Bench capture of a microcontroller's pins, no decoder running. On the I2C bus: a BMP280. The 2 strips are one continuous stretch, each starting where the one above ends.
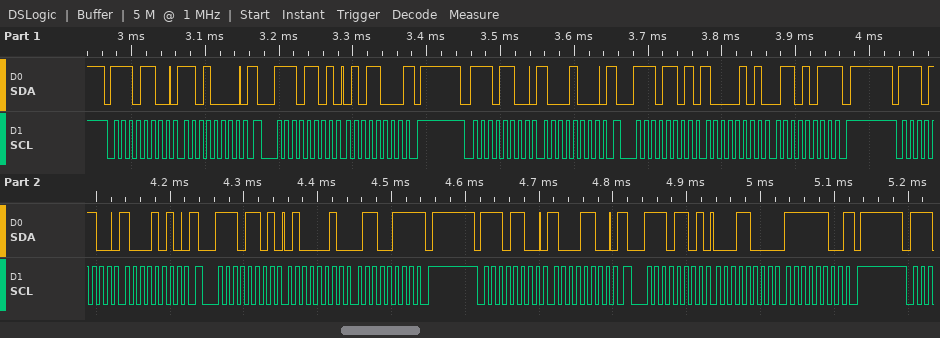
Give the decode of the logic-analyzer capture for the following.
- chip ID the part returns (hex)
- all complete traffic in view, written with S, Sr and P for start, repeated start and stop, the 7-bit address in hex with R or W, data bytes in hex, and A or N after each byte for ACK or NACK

0x58
S 76W A D0 A Sr 76R A 58 N P S 76W A 88 A Sr 76R A 85 A 6B N P S 76W A 8A A Sr 76R A 42 A 67 N P S 76W A 8C A Sr 76R A 18 A FC N P
